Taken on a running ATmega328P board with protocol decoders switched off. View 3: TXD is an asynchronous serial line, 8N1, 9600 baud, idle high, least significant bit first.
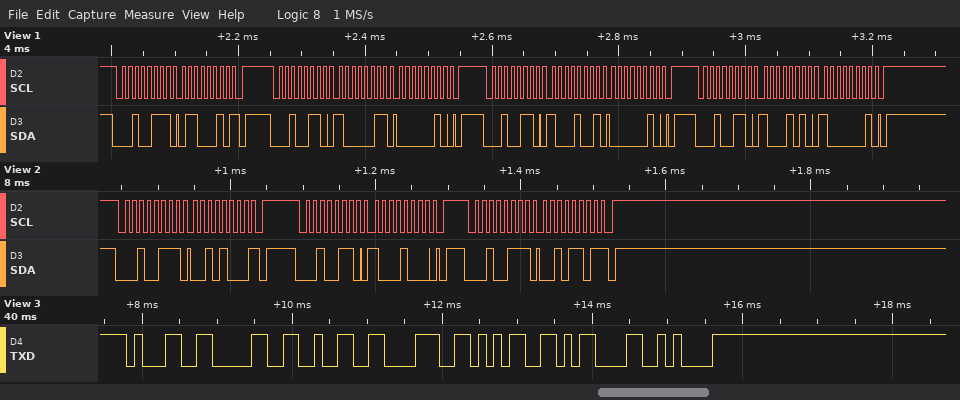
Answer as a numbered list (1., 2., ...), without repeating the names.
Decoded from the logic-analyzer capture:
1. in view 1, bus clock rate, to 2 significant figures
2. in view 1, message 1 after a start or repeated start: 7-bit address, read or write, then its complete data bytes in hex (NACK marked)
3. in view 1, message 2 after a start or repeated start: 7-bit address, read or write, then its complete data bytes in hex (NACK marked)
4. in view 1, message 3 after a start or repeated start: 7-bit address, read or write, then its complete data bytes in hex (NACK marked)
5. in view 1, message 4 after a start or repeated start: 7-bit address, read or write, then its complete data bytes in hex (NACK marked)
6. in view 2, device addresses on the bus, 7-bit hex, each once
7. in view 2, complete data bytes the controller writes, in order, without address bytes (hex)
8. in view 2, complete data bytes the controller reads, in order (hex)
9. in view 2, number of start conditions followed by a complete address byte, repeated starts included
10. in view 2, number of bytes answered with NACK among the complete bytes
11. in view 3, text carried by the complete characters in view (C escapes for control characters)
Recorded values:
1. 100 kHz
2. 0x13 read: 62 NACK
3. 0x13 write: 83 02
4. 0x13 write: 89 02
5. 0x13 write: 8A 81
6. 0x13
7. 88
8. 28 2D
9. 3
10. 2
11. "10285\r\n"
